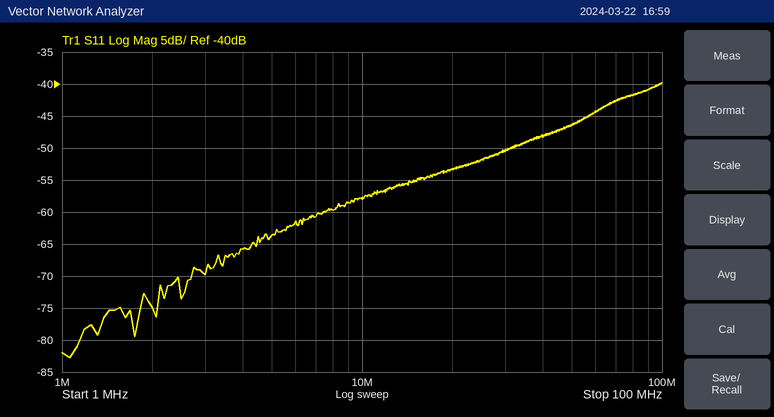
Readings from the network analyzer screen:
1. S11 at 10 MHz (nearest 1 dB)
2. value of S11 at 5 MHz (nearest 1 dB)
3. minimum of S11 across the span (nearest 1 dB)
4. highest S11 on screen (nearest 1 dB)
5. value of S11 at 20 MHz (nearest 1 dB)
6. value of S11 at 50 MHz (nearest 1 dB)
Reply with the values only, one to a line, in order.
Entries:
-58 dB
-64 dB
-83 dB
-40 dB
-53 dB
-46 dB
